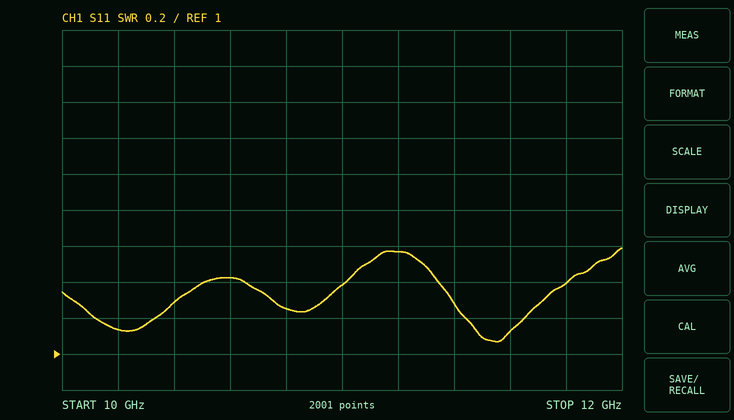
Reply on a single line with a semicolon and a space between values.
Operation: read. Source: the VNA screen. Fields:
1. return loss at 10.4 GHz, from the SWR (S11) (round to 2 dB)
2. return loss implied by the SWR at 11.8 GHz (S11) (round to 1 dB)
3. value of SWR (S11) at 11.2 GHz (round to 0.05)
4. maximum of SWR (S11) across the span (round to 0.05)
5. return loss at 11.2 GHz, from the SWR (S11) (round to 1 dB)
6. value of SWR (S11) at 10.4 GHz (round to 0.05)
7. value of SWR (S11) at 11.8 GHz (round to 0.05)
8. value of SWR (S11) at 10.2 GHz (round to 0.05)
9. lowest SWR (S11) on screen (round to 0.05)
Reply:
18 dB; 16 dB; 1.55; 1.60; 13 dB; 1.30; 1.40; 1.15; 1.05
